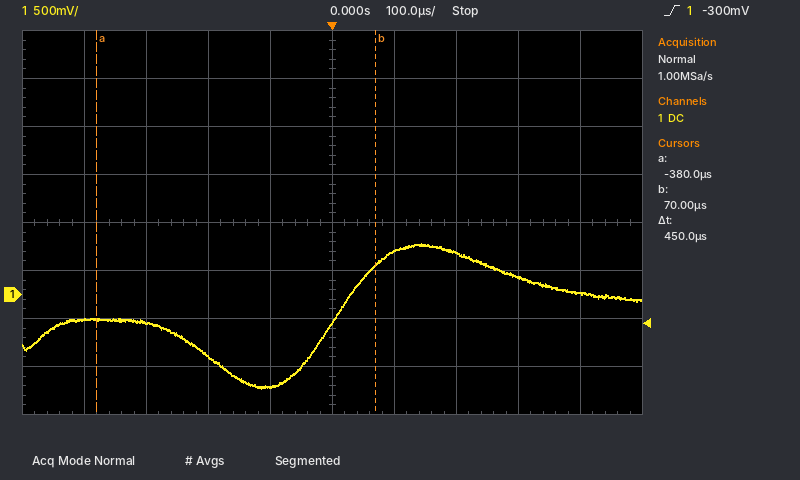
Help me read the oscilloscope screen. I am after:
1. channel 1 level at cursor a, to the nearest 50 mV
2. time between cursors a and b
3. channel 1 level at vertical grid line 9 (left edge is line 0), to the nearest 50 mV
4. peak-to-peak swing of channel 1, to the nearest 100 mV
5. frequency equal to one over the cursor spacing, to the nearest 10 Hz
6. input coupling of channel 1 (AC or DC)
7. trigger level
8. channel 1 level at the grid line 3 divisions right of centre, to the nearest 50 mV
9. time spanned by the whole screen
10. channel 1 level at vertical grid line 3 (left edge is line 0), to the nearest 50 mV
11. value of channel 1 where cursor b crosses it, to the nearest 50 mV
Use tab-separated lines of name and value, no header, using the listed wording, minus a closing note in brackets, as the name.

channel 1 level at cursor a, to the nearest 50 mV	-250 mV
time between cursors a and b	450 µs
channel 1 level at vertical grid line 9 (left edge is line 0), to the nearest 50 mV	0 mV
peak-to-peak swing of channel 1, to the nearest 100 mV	1.50 V
frequency equal to one over the cursor spacing, to the nearest 10 Hz	2.22 kHz
input coupling of channel 1	DC
trigger level	-300 mV
channel 1 level at the grid line 3 divisions right of centre, to the nearest 50 mV	200 mV
time spanned by the whole screen	1 ms
channel 1 level at vertical grid line 3 (left edge is line 0), to the nearest 50 mV	-650 mV
value of channel 1 where cursor b crosses it, to the nearest 50 mV	300 mV
